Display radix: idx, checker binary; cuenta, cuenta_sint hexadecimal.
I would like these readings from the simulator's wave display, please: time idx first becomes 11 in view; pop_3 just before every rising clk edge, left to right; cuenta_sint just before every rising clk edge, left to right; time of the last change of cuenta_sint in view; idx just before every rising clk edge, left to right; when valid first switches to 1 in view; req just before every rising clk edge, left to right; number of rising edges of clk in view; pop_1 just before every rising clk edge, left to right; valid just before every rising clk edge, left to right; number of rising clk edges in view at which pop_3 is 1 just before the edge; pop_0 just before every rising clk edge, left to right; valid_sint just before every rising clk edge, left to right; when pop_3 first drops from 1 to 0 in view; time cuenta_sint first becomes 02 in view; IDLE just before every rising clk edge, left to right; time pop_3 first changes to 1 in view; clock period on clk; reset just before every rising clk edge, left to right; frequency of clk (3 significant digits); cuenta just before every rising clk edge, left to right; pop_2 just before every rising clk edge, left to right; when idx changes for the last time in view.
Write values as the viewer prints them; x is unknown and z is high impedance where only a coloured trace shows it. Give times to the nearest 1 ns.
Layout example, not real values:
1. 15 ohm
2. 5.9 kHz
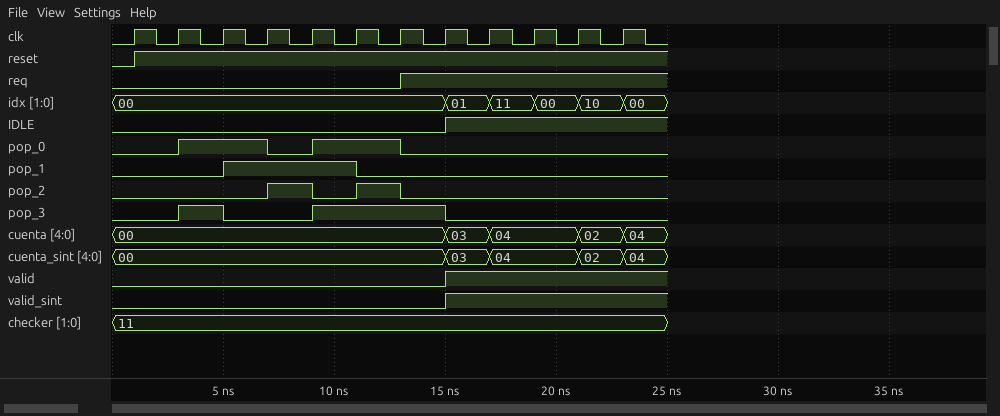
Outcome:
1. 17 ns
2. 0 0 1 0 0 1 1 1 0 0 0 0
3. 00, 00, 00, 00, 00, 00, 00, 00, 03, 04, 04, 02
4. 23 ns
5. 00, 00, 00, 00, 00, 00, 00, 00, 01, 11, 00, 10
6. 15 ns
7. 0 0 0 0 0 0 0 1 1 1 1 1
8. 12
9. 0 0 0 1 1 1 0 0 0 0 0 0
10. 0 0 0 0 0 0 0 0 1 1 1 1
11. 4
12. 0 0 1 1 0 1 1 0 0 0 0 0
13. 0 0 0 0 0 0 0 0 1 1 1 1
14. 5 ns
15. 21 ns
16. 0 0 0 0 0 0 0 0 1 1 1 1
17. 3 ns
18. 2 ns
19. 0 1 1 1 1 1 1 1 1 1 1 1
20. 500 MHz
21. 00, 00, 00, 00, 00, 00, 00, 00, 03, 04, 04, 02
22. 0 0 0 0 1 0 1 0 0 0 0 0
23. 23 ns
